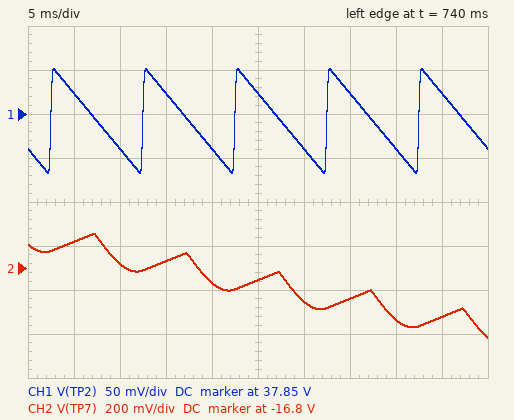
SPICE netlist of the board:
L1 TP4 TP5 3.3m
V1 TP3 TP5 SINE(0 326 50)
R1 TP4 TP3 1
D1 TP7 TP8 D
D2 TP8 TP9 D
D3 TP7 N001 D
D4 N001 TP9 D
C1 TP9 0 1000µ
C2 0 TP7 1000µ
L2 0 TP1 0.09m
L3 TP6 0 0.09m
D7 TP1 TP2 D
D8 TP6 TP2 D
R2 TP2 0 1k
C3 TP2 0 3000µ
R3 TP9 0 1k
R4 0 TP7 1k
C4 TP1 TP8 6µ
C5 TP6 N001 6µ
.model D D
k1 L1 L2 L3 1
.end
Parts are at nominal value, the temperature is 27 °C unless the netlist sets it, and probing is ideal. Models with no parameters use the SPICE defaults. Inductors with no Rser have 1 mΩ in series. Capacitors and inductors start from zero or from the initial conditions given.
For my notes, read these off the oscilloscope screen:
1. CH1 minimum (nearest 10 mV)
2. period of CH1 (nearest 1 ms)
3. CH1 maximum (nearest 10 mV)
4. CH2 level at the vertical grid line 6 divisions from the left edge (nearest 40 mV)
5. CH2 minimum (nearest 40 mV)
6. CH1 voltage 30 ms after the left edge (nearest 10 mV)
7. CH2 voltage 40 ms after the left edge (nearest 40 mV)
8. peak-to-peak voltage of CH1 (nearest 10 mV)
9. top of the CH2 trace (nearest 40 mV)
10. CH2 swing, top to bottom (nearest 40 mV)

37.78 V
10 ms
37.90 V
-16.96 V
-17.12 V
37.81 V
-17.04 V
120 mV
-16.64 V
480 mV
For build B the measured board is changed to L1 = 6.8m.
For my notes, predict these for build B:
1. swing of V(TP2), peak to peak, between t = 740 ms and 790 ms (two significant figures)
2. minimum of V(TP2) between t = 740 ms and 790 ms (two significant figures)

100 mV
33 V
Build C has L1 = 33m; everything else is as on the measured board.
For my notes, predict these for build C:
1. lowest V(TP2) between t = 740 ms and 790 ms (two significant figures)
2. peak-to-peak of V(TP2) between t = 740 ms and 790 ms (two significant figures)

16 V
50 mV
